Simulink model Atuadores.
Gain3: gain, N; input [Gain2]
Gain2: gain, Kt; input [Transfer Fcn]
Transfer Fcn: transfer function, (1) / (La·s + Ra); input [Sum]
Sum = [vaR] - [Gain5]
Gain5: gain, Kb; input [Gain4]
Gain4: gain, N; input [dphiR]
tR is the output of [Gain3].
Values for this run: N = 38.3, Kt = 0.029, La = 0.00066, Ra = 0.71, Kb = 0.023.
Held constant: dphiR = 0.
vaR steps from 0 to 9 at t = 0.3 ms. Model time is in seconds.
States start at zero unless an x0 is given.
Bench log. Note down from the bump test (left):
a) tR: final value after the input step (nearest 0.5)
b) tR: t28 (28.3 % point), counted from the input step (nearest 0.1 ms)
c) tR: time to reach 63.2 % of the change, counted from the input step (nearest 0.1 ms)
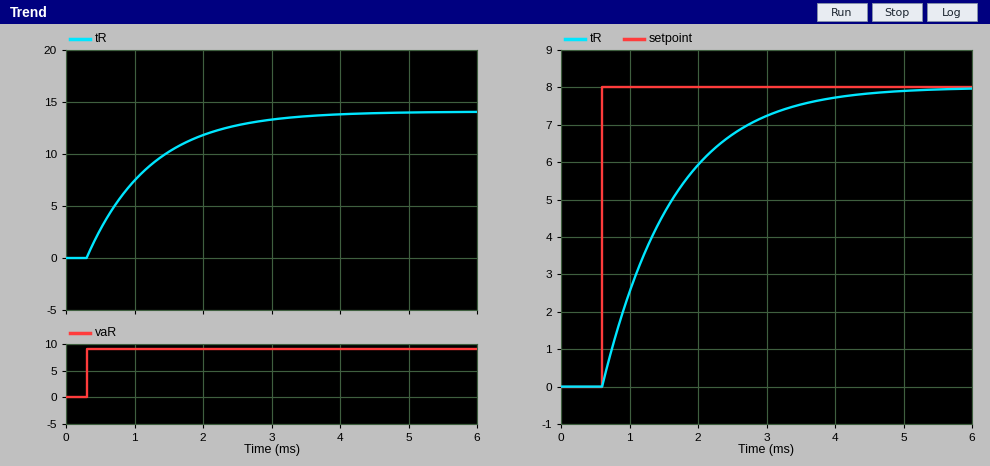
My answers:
14.0
0.3 ms
0.9 ms
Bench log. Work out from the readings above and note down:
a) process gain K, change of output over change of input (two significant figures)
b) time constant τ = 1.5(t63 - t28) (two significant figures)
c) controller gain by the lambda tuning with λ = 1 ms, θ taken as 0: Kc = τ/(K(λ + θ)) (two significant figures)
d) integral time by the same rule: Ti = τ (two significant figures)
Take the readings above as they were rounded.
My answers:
1.6
0.90 ms
0.56
0.90 ms
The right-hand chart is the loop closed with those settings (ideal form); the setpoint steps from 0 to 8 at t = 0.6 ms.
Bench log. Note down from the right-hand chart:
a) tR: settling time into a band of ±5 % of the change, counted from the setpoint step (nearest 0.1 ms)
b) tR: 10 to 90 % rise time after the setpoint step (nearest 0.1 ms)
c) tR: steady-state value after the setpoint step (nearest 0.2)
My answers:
3.0 ms
2.2 ms
8.0
